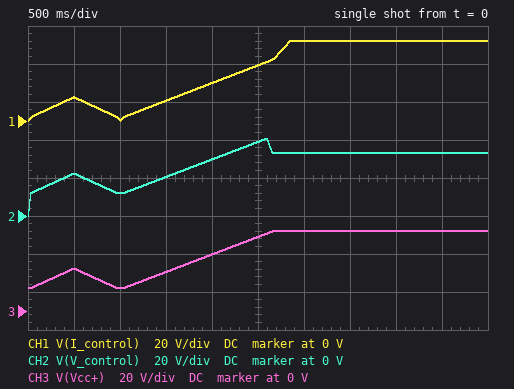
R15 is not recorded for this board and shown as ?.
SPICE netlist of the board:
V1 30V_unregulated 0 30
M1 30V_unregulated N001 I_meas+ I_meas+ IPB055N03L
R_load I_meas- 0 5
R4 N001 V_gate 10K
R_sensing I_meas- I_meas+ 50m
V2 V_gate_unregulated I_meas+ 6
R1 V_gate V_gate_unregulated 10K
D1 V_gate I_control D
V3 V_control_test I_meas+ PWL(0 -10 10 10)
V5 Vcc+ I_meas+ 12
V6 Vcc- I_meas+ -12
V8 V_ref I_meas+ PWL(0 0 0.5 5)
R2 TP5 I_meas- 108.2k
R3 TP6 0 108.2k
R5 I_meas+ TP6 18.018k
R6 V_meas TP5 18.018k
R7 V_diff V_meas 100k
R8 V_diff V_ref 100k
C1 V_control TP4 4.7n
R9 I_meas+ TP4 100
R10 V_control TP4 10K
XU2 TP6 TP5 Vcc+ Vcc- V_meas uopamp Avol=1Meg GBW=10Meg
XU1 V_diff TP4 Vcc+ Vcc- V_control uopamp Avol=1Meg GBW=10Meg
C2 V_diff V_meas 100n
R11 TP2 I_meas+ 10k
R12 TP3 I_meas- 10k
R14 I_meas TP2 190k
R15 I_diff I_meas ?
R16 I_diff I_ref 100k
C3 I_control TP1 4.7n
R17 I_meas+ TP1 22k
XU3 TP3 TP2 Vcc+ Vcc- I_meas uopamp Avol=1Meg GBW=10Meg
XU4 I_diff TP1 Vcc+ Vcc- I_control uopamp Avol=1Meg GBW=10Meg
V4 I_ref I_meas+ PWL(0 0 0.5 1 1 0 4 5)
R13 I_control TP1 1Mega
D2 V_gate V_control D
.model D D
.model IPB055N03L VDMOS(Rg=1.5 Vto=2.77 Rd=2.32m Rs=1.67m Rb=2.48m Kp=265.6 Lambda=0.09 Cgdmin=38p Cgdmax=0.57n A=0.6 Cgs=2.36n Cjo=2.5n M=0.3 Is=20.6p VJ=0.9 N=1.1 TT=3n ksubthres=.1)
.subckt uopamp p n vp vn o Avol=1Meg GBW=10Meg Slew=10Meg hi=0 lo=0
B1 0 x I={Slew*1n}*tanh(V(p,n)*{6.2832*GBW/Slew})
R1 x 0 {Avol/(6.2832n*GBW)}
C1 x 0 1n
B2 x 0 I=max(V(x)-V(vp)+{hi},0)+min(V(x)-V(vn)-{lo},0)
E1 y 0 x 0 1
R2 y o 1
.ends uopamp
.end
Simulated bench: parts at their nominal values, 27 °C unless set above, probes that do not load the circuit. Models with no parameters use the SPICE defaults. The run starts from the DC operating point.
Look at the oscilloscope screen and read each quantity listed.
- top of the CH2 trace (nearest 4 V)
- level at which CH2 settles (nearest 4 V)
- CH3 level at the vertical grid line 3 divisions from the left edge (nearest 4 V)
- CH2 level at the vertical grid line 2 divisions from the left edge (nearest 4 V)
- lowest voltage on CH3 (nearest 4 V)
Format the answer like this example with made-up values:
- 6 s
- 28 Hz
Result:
- 40 V
- 32 V
- 20 V
- 12 V
- 12 V
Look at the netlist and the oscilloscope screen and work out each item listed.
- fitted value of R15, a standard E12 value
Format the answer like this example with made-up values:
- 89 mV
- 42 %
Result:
- 220 kΩ
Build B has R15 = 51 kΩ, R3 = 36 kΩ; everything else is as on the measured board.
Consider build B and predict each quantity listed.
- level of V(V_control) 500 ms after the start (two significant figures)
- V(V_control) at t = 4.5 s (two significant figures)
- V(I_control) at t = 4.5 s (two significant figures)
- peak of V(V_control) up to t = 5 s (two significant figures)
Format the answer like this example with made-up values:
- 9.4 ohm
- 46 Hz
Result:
- 14 V
- 20 V
- 15 V
- 24 V
